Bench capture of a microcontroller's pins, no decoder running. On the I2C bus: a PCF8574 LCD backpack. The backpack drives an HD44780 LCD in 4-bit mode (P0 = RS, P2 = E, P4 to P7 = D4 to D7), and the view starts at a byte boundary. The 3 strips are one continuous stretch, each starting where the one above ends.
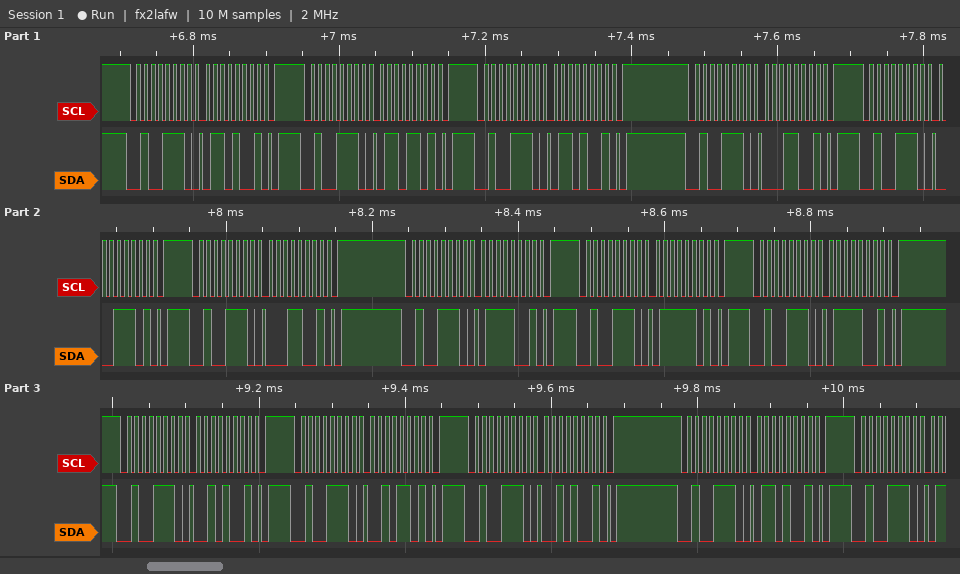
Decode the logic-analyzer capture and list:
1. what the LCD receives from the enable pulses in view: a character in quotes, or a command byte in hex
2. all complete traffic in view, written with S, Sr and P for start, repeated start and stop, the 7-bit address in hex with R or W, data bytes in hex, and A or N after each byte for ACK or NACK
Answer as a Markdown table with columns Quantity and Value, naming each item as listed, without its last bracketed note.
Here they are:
| Quantity | Value |
|---|---|
| what the LCD receives from the enable pulses in view: a character in quotes, or a command byte in hex | 'a' 'r' |
| all complete traffic in view, written with S, Sr and P for start, repeated start and stop, the 7-bit address in hex with R or W, data bytes in hex, and A or N after each byte for ACK or NACK | S 27W A 69 A P S 27W A 6D A P S 27W A 69 A P S 27W A 19 A P S 27W A 1D A P S 27W A 19 A P S 27W A 79 A P S 27W A 7D A P S 27W A 79 A P S 27W A 29 A P S 27W A 2D A P S 27W A 29 A P S 27W A 69 A P S 27W A |
